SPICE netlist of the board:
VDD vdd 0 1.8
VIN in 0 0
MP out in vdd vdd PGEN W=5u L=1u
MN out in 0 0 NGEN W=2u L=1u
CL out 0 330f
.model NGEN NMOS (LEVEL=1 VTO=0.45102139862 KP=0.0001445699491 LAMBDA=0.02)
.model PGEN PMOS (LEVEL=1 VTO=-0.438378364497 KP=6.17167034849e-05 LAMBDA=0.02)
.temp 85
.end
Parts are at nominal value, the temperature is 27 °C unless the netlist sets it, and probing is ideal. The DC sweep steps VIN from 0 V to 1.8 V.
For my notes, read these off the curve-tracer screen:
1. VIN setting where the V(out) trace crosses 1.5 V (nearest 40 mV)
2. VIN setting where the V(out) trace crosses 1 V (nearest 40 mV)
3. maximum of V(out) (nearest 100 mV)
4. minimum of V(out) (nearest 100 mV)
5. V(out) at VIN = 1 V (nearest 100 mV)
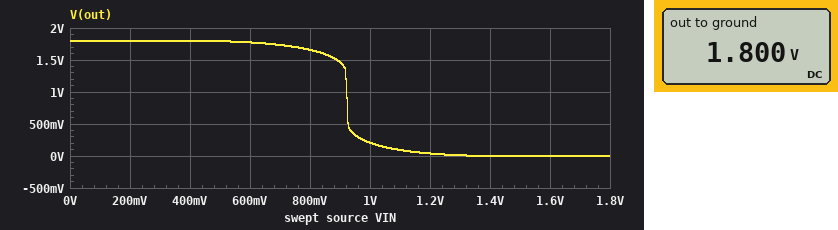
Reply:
880 mV
920 mV
1.8 V
0 V
200 mV
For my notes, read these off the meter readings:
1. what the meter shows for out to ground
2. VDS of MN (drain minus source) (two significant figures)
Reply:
1.800 V
1.8 V
